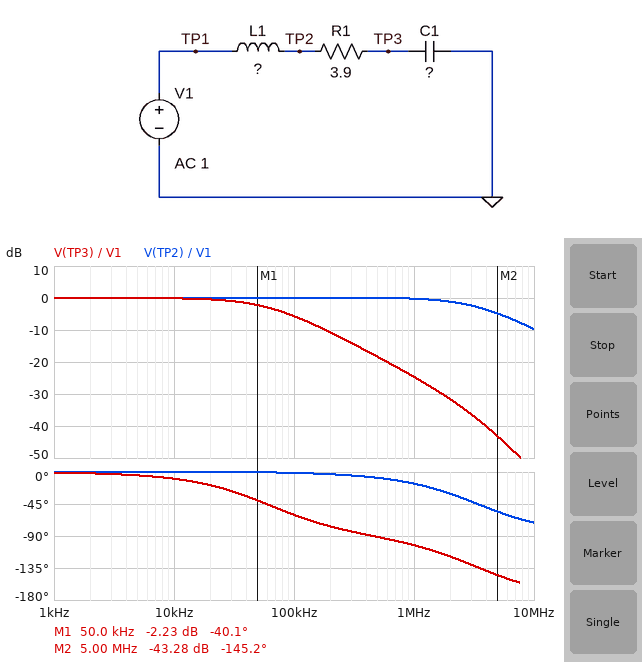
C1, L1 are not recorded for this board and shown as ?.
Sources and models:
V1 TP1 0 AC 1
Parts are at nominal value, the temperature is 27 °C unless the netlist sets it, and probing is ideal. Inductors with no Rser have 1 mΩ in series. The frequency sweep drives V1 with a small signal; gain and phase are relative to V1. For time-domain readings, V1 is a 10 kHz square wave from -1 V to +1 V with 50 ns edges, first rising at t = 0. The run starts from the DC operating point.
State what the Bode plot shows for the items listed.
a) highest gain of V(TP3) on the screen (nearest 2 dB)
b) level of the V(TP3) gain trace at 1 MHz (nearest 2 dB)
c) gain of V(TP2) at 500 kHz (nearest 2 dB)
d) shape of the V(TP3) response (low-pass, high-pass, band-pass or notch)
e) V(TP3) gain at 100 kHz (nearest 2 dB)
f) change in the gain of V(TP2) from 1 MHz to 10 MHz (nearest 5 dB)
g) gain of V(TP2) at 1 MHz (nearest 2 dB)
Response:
0 dB
-24 dB
0 dB
low-pass
-6 dB
-10 dB
0 dB
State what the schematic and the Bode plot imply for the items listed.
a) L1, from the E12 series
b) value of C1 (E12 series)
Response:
180 nH
680 nF
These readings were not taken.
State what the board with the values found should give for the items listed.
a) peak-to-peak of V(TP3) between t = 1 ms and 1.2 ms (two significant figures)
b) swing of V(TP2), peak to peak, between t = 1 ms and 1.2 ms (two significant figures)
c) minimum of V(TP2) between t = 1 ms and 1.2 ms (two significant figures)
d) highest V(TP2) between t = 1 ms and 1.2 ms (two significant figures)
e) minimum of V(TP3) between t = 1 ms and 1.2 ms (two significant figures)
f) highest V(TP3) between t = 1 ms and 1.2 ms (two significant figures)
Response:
2.0 V
2.1 V
-1.0 V
1.0 V
-1.0 V
1.0 V
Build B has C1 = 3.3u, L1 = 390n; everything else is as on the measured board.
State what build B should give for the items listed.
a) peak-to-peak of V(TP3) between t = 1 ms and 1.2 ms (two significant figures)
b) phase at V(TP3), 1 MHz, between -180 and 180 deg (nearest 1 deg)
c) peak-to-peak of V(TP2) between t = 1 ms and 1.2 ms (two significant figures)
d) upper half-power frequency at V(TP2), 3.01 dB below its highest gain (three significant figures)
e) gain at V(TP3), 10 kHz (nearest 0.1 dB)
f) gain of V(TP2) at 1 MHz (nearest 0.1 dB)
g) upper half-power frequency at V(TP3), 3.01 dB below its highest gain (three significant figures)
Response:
1.9 V
-122 deg
2.0 V
1.58 MHz
-2.2 dB
-1.4 dB
12.5 kHz
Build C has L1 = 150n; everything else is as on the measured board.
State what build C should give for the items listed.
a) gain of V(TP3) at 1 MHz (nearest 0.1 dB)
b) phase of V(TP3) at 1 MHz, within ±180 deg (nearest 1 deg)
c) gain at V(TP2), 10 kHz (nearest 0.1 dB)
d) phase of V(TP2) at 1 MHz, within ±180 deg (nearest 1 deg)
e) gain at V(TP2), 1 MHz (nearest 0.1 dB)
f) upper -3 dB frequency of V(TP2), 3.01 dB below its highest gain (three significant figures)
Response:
-24.6 dB
-100 deg
0 dB
-14 deg
-0.1 dB
4.10 MHz
